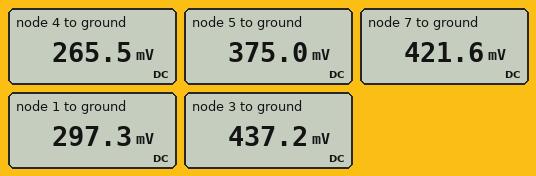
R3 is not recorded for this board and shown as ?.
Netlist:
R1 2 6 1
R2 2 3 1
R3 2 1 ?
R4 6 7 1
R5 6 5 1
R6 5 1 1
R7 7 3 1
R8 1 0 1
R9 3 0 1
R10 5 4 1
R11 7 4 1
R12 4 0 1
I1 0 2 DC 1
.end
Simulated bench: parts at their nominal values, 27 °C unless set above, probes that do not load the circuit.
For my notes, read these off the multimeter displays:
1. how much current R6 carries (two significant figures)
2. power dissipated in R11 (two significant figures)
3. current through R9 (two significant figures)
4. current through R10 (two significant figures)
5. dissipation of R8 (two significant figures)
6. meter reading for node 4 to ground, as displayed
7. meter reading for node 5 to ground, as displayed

78 mA
24 mW
440 mA
110 mA
88 mW
265.5 mV
375.0 mV
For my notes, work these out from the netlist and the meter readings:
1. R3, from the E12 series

2.7 Ω
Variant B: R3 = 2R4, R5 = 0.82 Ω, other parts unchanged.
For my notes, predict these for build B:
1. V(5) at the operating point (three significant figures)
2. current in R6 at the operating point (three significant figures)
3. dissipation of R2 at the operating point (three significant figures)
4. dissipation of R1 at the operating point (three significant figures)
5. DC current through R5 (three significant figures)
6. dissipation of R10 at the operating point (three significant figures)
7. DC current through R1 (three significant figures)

384 mV
75.3 mA
195 mW
106 mW
194 mA
14.1 mW
325 mA
